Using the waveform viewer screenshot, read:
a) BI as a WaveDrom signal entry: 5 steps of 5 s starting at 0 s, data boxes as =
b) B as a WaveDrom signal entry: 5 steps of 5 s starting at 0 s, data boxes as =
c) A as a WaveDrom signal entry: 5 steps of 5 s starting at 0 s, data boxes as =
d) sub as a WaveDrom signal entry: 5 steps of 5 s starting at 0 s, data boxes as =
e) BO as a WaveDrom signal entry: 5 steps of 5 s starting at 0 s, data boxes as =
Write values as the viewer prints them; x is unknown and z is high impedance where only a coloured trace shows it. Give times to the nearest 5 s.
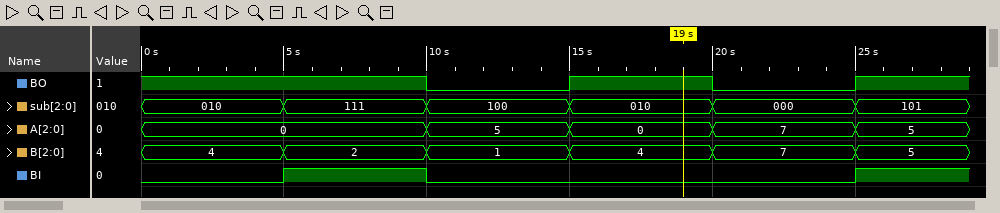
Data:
{name: 'BI', wave: '010..'}
{name: 'B', wave: '=====', data: '4 2 1 4 7'}
{name: 'A', wave: '=.===', data: '0 5 0 7'}
{name: 'sub', wave: '=====', data: '010 111 100 010 000'}
{name: 'BO', wave: '1.010'}
